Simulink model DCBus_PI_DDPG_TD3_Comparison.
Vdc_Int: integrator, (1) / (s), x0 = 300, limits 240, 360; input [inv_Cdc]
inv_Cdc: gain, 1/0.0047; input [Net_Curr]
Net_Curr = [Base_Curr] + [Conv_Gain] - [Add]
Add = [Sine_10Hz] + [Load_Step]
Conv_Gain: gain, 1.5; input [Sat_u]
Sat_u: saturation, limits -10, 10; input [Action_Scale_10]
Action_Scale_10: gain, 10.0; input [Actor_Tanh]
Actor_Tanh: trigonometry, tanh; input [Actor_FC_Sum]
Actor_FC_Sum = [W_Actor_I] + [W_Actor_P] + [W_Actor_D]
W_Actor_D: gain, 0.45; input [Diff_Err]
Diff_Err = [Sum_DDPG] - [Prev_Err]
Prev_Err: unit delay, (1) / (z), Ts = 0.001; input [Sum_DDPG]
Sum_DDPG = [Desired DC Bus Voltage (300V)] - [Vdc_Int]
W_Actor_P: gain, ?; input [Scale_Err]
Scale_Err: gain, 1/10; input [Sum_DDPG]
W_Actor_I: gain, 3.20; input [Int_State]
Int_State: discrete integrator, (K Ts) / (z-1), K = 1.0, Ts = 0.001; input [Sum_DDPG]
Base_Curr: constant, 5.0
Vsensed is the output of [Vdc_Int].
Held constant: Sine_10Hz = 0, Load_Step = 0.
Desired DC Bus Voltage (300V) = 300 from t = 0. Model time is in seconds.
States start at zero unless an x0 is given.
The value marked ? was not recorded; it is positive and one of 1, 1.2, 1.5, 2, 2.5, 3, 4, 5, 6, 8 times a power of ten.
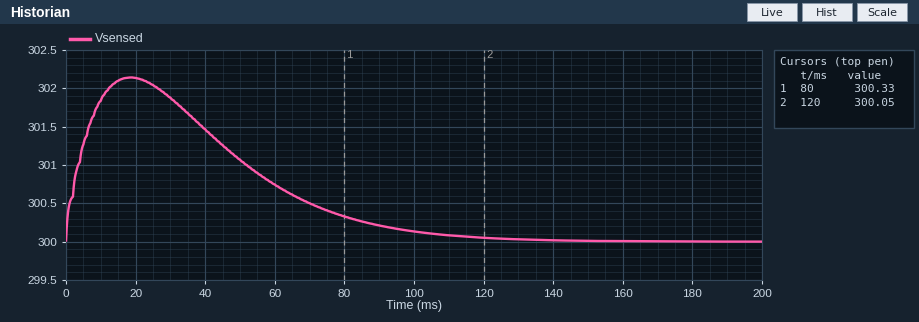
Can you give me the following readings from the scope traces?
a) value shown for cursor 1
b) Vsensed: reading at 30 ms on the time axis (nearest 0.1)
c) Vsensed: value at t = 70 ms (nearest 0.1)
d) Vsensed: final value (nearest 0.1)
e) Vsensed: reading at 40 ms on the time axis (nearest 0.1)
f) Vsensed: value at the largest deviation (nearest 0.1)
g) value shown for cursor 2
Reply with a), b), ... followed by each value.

a) 300.33
b) 301.9
c) 300.5
d) 300.0
e) 301.5
f) 302.1
g) 300.05
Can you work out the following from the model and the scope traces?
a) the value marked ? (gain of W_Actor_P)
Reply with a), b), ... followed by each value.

a) 1.2
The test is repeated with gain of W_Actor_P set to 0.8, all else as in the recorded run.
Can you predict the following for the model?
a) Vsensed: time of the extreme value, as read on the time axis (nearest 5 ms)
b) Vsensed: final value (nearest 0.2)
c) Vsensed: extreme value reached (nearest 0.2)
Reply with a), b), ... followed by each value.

a) 20 ms
b) 300.0
c) 302.8
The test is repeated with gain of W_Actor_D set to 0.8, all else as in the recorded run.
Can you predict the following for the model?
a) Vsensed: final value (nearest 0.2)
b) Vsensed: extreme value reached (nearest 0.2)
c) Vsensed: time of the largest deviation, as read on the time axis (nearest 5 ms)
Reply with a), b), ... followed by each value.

a) 300.0
b) 302.0
c) 25 ms
